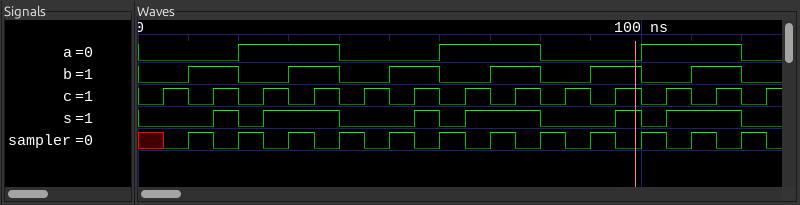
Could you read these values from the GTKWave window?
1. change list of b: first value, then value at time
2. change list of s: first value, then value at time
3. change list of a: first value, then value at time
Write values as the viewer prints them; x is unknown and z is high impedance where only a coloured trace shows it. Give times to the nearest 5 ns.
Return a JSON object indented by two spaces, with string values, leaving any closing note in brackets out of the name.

{
  "change list of b: first value, then value at time": "0, 1 at 10 ns, 0 at 20 ns, 1 at 30 ns, 0 at 40 ns, 1 at 50 ns, 0 at 60 ns, 1 at 70 ns, 0 at 80 ns, 1 at 90 ns, 0 at 100 ns, 1 at 110 ns, 0 at 120 ns",
  "change list of s: first value, then value at time": "0, 1 at 15 ns, 0 at 20 ns, 1 at 25 ns, 0 at 40 ns, 1 at 55 ns, 0 at 60 ns, 1 at 65 ns, 0 at 80 ns, 1 at 95 ns, 0 at 100 ns, 1 at 105 ns, 0 at 120 ns",
  "change list of a: first value, then value at time": "0, 1 at 20 ns, 0 at 40 ns, 1 at 60 ns, 0 at 80 ns, 1 at 100 ns, 0 at 120 ns"
}
